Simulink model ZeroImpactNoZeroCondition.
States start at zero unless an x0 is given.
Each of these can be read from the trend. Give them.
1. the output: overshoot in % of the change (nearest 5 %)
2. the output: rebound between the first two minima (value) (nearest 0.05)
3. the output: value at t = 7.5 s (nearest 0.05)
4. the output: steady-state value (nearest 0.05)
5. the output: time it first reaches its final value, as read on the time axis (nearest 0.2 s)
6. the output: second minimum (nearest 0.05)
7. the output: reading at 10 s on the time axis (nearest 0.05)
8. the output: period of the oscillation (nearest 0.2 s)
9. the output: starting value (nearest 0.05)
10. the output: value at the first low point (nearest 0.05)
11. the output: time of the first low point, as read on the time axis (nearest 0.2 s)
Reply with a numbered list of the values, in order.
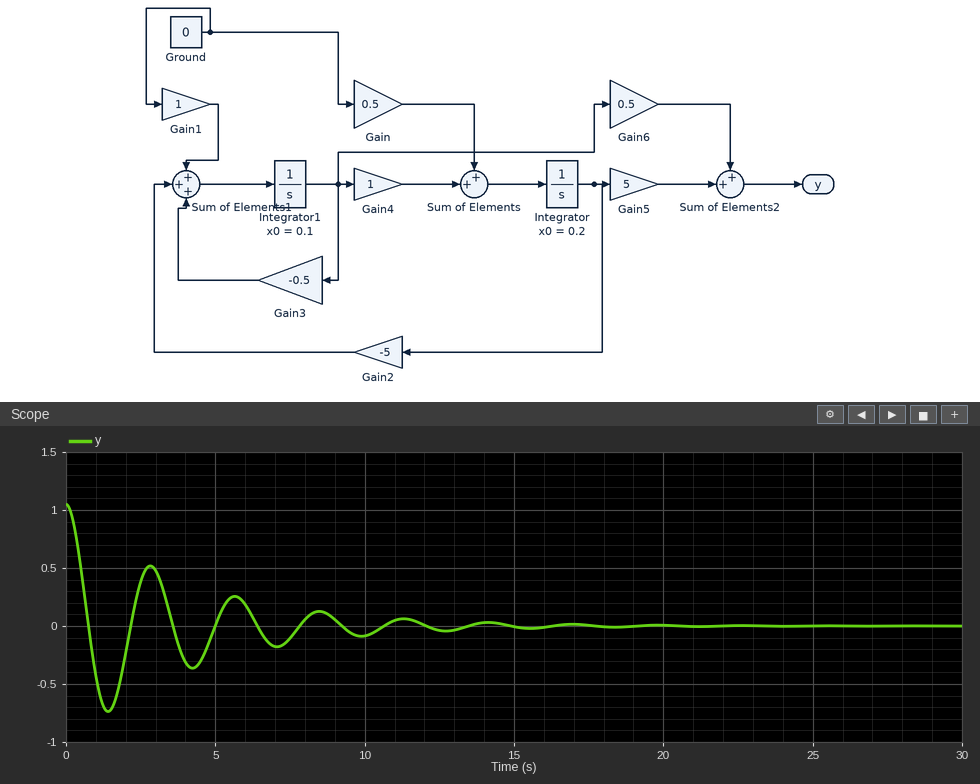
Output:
1. 70 %
2. 0.50
3. -0.10
4. 0.00
5. 0.8 s
6. -0.35
7. -0.10
8. 2.8 s
9. 1.05
10. -0.75
11. 1.4 s
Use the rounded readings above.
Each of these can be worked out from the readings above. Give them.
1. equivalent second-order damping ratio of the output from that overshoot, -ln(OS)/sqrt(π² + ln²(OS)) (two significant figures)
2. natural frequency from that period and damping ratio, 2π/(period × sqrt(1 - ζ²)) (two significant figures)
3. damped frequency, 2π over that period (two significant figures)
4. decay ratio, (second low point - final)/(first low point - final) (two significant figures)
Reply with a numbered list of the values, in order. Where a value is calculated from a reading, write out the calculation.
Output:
1. ln(0.7) = -0.357; 0.357 / sqrt(9.870 + 0.127) = 0.11
2. 2π / (2.8 × sqrt(1 - 0.11²)) = 2.3 rad/s
3. 2π / 2.8 = 2.2 rad/s
4. (-0.35 - 0) / (-0.75 - 0) = 0.47
